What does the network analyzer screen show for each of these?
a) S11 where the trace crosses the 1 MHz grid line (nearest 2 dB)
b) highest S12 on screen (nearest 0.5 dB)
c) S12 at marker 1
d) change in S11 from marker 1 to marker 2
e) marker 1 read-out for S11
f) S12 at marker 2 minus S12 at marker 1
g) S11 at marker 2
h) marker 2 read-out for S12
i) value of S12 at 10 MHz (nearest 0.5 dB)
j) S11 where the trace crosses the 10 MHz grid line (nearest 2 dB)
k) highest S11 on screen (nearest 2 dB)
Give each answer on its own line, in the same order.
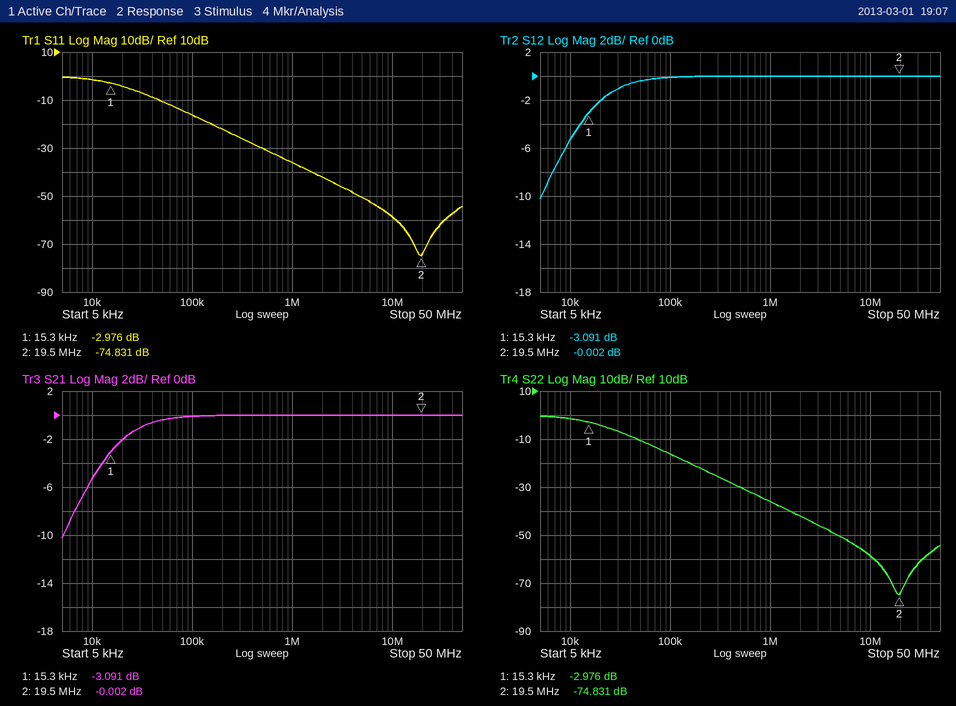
-36 dB
0.0 dB
-3.091 dB
-71.855 dB
-2.976 dB
3.089 dB
-74.831 dB
-0.002 dB
0.0 dB
-58 dB
0 dB
